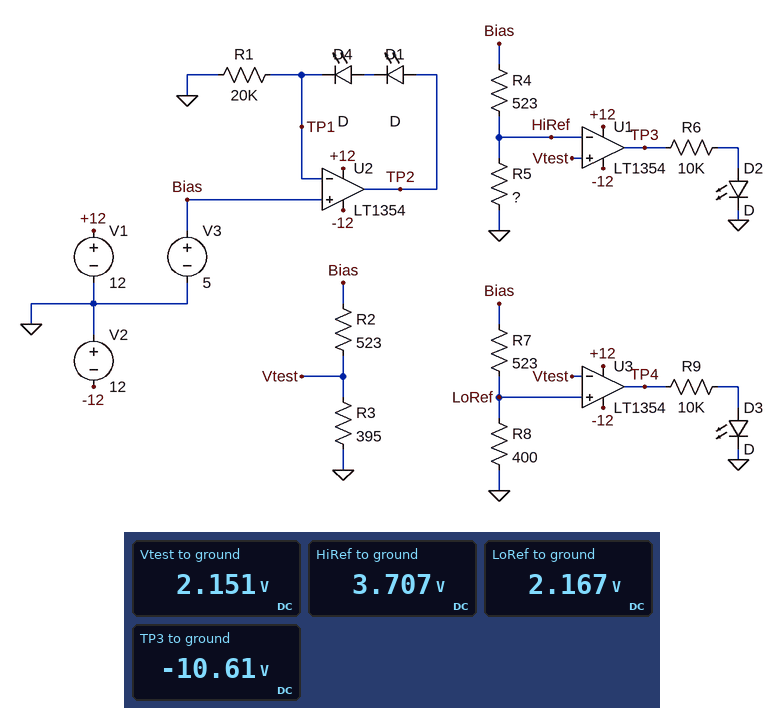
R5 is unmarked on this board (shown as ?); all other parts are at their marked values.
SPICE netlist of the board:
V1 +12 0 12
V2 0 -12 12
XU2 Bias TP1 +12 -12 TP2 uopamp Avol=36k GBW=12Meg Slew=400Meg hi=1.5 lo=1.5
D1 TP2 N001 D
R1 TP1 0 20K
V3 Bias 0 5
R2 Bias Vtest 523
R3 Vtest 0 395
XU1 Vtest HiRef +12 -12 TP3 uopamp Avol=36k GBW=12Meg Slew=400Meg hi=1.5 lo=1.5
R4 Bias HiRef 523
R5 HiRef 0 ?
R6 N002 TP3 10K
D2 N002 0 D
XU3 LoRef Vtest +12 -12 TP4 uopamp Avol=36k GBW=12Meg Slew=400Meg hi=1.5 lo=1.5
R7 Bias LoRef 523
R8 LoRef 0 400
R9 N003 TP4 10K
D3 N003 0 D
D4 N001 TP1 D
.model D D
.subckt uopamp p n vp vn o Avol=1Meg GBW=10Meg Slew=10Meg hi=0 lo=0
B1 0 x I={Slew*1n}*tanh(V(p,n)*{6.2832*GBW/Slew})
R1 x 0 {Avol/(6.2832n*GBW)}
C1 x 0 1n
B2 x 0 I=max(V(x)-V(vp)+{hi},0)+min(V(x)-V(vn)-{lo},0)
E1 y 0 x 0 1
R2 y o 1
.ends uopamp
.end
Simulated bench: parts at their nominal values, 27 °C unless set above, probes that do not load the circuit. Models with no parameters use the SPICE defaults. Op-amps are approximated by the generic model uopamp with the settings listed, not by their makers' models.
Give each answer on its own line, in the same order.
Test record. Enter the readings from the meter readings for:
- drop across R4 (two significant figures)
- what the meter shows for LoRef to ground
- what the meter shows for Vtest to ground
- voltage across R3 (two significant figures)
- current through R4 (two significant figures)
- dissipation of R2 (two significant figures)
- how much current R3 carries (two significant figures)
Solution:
1.3 V
2.167 V
2.151 V
2.2 V
2.5 mA
16 mW
5.4 mA
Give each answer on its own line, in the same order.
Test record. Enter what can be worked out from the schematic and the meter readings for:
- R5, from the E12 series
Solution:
1.5 kΩ
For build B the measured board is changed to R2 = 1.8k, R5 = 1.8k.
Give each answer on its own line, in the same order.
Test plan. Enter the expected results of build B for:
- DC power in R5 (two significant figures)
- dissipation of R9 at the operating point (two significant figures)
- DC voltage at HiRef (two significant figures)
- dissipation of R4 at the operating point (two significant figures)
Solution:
8.3 mW
9.9 mW
3.9 V
2.4 mW
